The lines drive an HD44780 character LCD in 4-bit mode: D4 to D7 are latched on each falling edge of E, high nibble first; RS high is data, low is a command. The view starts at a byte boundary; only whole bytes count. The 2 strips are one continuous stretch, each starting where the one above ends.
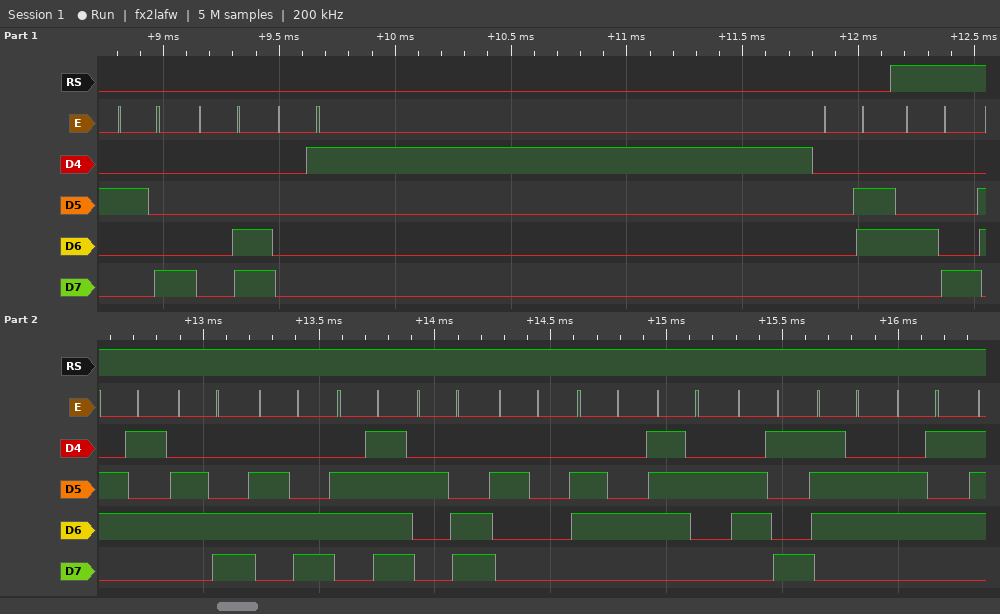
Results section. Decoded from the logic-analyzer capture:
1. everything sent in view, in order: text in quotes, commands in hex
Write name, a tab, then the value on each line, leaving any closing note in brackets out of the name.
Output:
everything sent in view, in order: text in quotes, commands in hex	0x28 0x0C 0x01 0x06 "Hello, drive"
